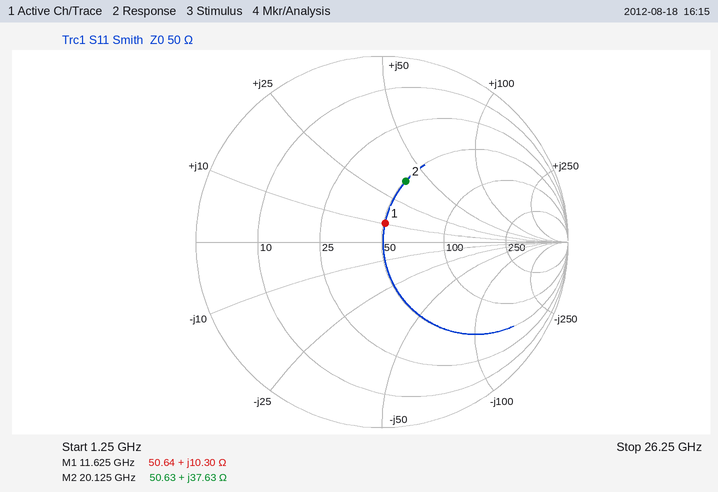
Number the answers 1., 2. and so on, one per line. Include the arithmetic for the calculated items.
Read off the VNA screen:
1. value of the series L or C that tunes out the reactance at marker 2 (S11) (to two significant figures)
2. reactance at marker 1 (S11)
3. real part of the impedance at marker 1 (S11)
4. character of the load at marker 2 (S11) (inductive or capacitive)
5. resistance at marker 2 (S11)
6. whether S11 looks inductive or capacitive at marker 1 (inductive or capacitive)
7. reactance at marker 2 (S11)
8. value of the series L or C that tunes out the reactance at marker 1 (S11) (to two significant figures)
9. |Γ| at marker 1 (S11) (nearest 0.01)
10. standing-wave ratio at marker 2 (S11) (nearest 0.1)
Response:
1. C = 1/(2π × 20.125 GHz × 37.63 Ω) ≈ 210 fF
2. +10.30 Ω
3. 50.64 Ω
4. inductive
5. 50.63 Ω
6. inductive
7. +37.63 Ω
8. C = 1/(2π × 11.625 GHz × 10.3 Ω) ≈ 1.3 pF
9. 0.10
10. 2.1
